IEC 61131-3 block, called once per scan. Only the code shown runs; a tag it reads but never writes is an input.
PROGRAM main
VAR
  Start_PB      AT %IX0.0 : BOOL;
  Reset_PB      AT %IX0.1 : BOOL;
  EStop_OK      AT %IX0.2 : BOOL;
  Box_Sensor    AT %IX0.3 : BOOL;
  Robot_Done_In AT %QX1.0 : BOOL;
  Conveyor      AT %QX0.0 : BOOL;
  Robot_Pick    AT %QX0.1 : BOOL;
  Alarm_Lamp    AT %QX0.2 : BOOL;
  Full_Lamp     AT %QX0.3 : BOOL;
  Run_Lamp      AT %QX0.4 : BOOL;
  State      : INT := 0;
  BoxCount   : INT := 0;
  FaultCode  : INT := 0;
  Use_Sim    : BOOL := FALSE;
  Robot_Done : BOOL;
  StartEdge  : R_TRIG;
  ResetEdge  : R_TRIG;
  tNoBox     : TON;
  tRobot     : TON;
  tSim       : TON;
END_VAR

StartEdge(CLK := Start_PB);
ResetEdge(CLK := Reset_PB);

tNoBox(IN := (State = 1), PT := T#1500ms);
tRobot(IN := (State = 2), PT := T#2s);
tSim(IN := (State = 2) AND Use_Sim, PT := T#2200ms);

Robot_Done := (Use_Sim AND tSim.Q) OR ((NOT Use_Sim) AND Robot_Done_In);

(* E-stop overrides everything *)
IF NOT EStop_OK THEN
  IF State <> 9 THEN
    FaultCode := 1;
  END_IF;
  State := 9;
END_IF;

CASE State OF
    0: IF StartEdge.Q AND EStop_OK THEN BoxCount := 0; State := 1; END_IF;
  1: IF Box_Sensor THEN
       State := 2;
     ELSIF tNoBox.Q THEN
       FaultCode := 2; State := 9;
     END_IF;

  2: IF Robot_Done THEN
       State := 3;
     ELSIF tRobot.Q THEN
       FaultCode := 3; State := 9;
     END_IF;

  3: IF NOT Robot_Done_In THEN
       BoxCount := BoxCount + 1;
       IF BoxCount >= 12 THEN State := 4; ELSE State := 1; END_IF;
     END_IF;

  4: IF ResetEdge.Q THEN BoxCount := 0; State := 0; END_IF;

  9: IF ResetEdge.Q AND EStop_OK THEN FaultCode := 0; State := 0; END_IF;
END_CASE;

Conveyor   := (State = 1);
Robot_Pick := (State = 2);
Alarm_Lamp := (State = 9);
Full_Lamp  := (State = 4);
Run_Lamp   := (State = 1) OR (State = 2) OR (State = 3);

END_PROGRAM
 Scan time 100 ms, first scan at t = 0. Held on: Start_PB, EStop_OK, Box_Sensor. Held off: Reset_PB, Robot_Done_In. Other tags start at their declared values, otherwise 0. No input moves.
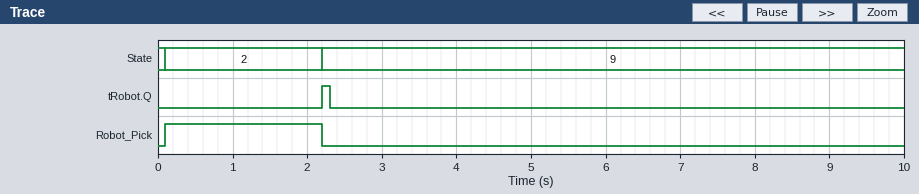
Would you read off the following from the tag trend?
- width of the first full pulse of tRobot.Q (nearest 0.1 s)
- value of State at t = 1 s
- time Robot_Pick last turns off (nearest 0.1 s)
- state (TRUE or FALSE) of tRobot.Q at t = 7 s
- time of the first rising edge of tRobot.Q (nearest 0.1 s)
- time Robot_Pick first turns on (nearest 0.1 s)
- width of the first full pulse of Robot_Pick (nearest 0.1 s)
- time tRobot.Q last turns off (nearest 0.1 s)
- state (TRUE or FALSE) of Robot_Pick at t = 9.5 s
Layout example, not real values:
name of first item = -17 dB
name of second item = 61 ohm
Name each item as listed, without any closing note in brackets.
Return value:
width of the first full pulse of tRobot.Q = 0.1 s
value of State at t = 1 s = 2
time Robot_Pick last turns off = 2.2 s
state (TRUE or FALSE) of tRobot.Q at t = 7 s = FALSE
time of the first rising edge of tRobot.Q = 2.2 s
time Robot_Pick first turns on = 0.1 s
width of the first full pulse of Robot_Pick = 2.1 s
time tRobot.Q last turns off = 2.3 s
state (TRUE or FALSE) of Robot_Pick at t = 9.5 s = FALSE
